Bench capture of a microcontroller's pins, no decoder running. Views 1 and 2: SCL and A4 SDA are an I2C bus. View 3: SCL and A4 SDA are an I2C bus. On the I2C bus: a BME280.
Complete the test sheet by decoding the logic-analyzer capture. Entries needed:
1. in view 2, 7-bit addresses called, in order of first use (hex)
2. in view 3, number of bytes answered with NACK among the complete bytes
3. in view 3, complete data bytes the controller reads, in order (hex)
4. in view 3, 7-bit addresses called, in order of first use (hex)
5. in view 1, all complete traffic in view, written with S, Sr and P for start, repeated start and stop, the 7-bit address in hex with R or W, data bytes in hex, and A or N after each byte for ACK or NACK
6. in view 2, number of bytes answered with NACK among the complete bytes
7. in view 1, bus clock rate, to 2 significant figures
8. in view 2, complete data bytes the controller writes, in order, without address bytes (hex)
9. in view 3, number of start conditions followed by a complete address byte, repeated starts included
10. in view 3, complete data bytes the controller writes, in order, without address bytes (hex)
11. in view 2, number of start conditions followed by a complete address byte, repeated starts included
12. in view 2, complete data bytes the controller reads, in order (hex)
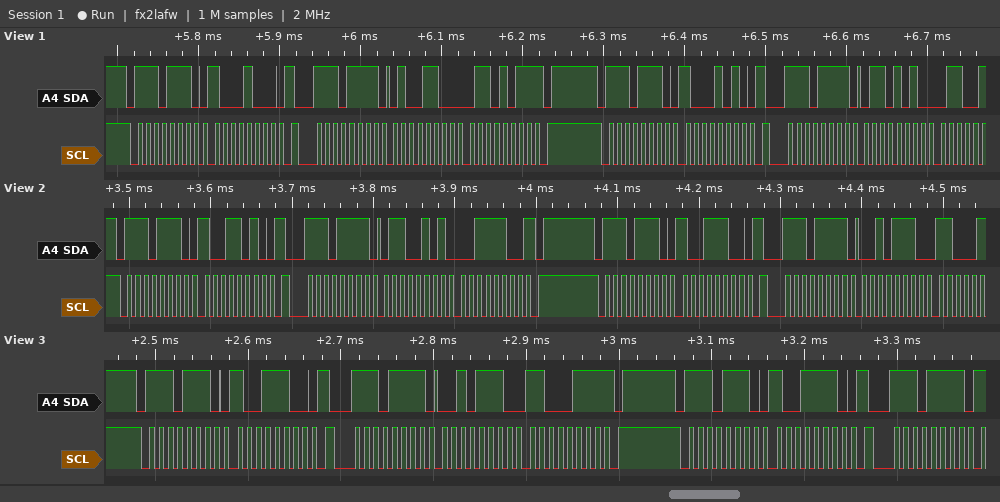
0x77
1
2E C7
0x77
S 77W A 88 A Sr 77R A 4C A 6B N P S 77W A 8A A Sr 77R A 6A A
1
100 kHz
9A 9C
4
9C 9E
4
65 3C 2E
